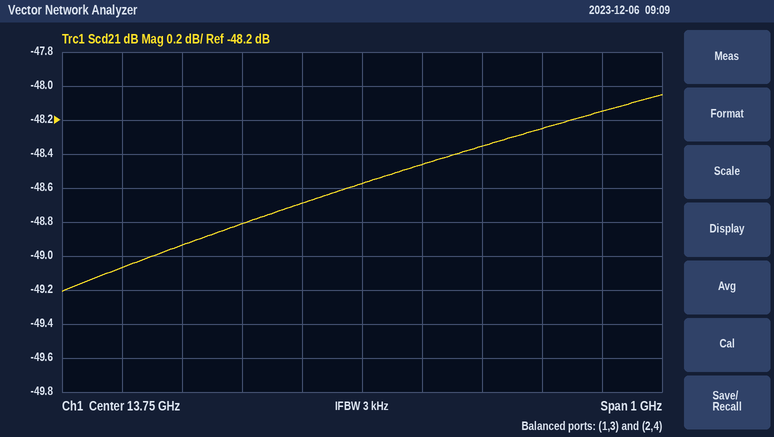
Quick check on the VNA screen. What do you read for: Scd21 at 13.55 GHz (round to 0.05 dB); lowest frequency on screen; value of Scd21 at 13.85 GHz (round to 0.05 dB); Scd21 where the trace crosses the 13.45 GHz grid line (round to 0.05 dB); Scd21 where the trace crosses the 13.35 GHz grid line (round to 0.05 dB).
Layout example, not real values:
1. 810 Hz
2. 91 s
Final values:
1. -48.80 dB
2. 13.25 GHz
3. -48.45 dB
4. -48.95 dB
5. -49.05 dB
